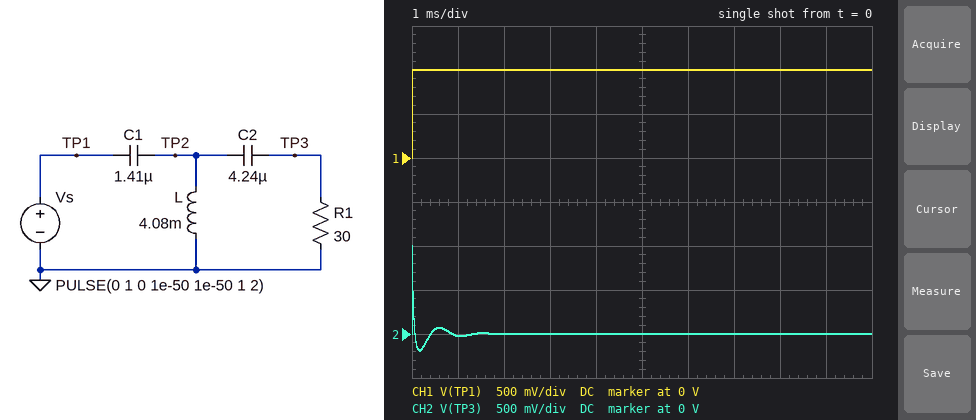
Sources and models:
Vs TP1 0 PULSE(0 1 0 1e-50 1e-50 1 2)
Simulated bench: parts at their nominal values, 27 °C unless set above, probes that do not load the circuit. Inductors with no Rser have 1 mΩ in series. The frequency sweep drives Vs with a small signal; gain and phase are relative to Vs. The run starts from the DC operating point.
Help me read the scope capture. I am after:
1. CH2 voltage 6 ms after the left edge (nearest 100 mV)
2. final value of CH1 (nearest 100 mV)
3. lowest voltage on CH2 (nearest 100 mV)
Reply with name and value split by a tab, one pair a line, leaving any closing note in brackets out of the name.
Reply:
CH2 voltage 6 ms after the left edge	0 V
final value of CH1	1.0 V
lowest voltage on CH2	-200 mV
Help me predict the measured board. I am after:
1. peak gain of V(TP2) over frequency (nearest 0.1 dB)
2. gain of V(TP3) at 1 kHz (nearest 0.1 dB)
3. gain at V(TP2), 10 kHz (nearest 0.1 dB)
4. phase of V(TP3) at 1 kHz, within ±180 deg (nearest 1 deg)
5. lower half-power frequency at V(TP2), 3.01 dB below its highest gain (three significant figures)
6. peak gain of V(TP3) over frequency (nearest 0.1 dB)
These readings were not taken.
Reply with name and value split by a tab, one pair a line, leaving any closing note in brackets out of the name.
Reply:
peak gain of V(TP2) over frequency	0 dB
gain of V(TP3) at 1 kHz	-10.7 dB
gain at V(TP2), 10 kHz	-0.6 dB
phase of V(TP3) at 1 kHz, within ±180 deg	-172 deg
lower half-power frequency at V(TP2), 3.01 dB below its highest gain	3.14 kHz
peak gain of V(TP3) over frequency	0 dB
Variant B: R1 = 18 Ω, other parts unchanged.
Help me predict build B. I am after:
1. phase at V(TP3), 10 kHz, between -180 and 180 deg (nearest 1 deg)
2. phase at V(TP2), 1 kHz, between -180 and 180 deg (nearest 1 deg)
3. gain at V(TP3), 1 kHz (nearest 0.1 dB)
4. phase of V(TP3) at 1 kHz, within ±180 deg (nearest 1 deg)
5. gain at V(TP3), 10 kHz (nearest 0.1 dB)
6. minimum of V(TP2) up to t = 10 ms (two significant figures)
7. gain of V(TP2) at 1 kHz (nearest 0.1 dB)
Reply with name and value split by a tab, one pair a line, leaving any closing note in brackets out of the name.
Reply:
phase at V(TP3), 10 kHz, between -180 and 180 deg	41 deg
phase at V(TP2), 1 kHz, between -180 and 180 deg	129 deg
gain at V(TP3), 1 kHz	-10.9 dB
phase of V(TP3) at 1 kHz, within ±180 deg	-166 deg
gain at V(TP3), 10 kHz	-2.0 dB
minimum of V(TP2) up to t = 10 ms	-170 mV
gain of V(TP2) at 1 kHz	-3.6 dB
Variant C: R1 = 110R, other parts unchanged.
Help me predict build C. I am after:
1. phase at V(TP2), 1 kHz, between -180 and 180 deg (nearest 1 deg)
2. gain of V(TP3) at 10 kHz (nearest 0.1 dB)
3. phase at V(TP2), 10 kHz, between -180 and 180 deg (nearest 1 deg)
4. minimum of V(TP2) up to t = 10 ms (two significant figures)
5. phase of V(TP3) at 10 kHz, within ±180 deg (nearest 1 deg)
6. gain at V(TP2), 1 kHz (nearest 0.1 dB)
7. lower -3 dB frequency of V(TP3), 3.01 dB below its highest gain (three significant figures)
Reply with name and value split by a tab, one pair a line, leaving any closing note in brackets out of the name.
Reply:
phase at V(TP2), 1 kHz, between -180 and 180 deg	163 deg
gain of V(TP3) at 10 kHz	0.3 dB
phase at V(TP2), 10 kHz, between -180 and 180 deg	6 deg
minimum of V(TP2) up to t = 10 ms	-510 mV
phase of V(TP3) at 10 kHz, within ±180 deg	8 deg
gain at V(TP2), 1 kHz	-10.2 dB
lower -3 dB frequency of V(TP3), 3.01 dB below its highest gain	1.73 kHz
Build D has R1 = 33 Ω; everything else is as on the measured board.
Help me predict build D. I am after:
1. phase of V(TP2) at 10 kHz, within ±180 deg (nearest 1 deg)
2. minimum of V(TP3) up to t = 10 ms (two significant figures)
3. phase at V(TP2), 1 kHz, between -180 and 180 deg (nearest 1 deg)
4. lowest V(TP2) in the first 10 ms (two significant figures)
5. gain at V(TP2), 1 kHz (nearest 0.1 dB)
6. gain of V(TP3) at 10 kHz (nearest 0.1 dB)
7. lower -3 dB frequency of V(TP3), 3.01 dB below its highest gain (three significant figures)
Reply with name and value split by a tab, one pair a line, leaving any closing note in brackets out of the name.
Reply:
phase of V(TP2) at 10 kHz, within ±180 deg	19 deg
minimum of V(TP3) up to t = 10 ms	-210 mV
phase at V(TP2), 1 kHz, between -180 and 180 deg	139 deg
lowest V(TP2) in the first 10 ms	-190 mV
gain at V(TP2), 1 kHz	-7.1 dB
gain of V(TP3) at 10 kHz	-0.5 dB
lower -3 dB frequency of V(TP3), 3.01 dB below its highest gain	3.08 kHz
